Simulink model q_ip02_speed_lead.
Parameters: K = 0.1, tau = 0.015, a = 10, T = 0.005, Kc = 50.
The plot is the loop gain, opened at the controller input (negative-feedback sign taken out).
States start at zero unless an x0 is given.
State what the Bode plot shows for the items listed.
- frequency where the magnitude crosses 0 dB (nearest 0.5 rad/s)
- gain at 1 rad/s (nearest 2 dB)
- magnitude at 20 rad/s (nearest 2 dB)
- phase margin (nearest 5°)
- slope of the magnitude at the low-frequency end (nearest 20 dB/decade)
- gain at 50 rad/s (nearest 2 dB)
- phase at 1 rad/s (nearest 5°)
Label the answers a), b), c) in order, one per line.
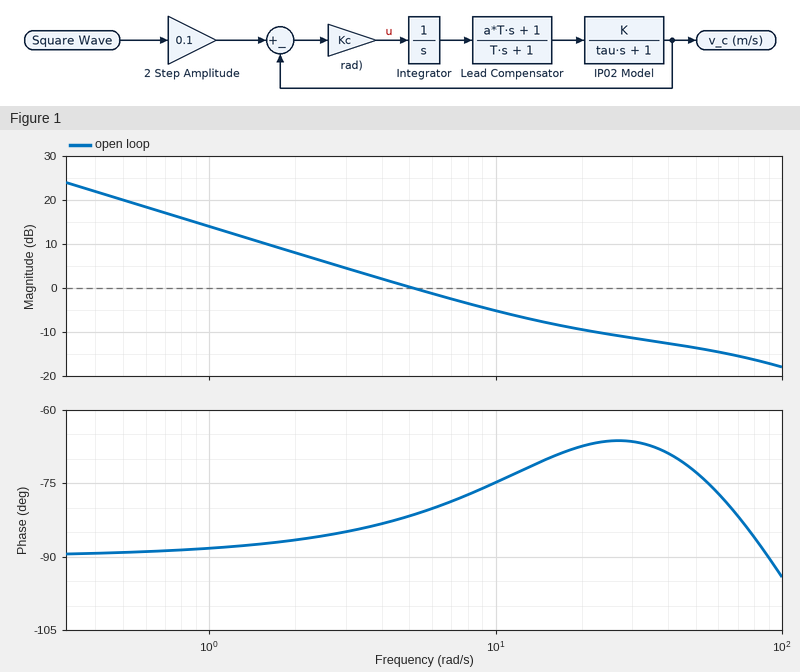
a) 5.0 rad/s
b) 14 dB
c) -10 dB
d) 100°
e) -20 dB/decade
f) -14 dB
g) -90°
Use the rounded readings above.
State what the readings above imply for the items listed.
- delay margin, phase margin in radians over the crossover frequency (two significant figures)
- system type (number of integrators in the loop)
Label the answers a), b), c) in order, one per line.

a) 0.35 s
b) 1
